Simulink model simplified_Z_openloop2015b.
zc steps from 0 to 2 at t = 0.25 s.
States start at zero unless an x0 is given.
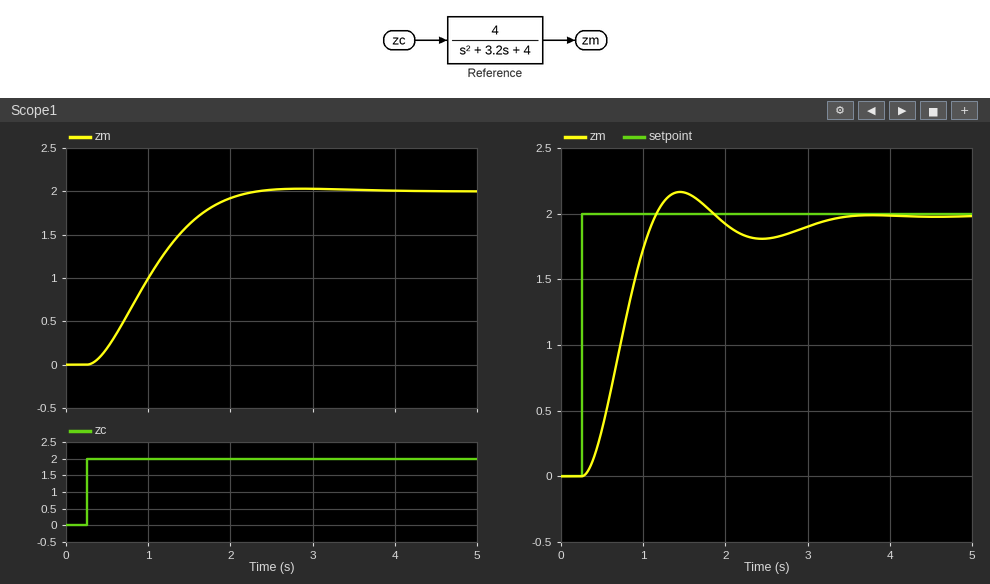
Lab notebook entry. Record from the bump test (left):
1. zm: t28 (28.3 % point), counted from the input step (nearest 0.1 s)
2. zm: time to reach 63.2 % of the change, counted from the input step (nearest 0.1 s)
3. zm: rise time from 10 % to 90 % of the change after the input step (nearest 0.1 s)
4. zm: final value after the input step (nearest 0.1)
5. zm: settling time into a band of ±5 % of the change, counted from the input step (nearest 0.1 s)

0.5 s
0.9 s
1.2 s
2.0
1.7 s
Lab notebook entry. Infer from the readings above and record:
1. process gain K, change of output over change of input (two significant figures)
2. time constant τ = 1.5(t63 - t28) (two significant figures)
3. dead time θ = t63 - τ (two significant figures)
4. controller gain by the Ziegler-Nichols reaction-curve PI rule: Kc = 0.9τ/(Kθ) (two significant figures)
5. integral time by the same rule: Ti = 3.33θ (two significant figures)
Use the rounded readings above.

1.0
0.60 s
0.30 s
1.8
1.00 s
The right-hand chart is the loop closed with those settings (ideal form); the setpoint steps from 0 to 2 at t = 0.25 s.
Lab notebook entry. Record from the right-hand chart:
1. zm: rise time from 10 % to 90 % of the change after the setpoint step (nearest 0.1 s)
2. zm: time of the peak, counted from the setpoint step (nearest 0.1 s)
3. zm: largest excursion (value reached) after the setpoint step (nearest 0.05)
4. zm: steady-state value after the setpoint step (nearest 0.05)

0.6 s
1.2 s
2.15
2.00
